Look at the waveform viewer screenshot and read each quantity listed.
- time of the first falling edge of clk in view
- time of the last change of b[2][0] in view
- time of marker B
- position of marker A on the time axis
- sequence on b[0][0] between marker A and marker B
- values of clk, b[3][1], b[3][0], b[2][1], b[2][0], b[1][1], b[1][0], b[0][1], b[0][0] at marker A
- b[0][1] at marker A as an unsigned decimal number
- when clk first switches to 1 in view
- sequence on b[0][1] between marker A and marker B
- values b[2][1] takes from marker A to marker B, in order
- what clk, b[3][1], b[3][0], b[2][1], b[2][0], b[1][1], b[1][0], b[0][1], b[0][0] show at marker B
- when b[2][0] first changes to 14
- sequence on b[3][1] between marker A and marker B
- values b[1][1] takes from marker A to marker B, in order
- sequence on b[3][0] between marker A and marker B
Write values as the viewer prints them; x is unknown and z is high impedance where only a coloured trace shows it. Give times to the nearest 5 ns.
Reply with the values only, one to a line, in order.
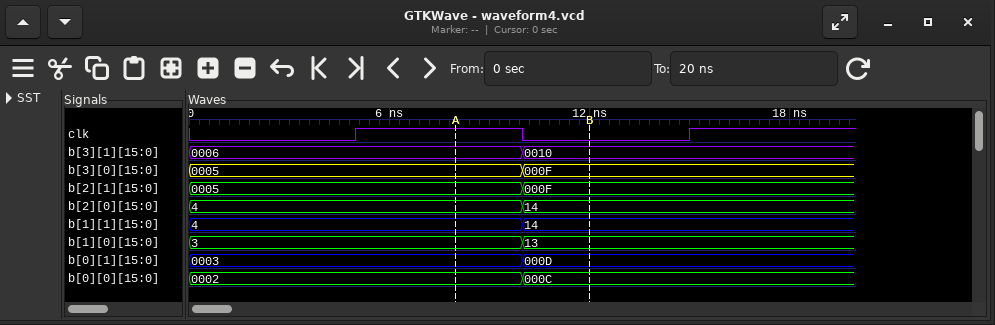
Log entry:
10 ns
10 ns
10 ns
10 ns
0002, 000C
clk=1, b[3][1]=0006, b[3][0]=0005, b[2][1]=0005, b[2][0]=4, b[1][1]=4, b[1][0]=3, b[0][1]=0003, b[0][0]=0002
3
5 ns
0003, 000D
0005, 000F
clk=0, b[3][1]=0010, b[3][0]=000F, b[2][1]=000F, b[2][0]=14, b[1][1]=14, b[1][0]=13, b[0][1]=000D, b[0][0]=000C
10 ns
0006, 0010
4, 14
0005, 000F
